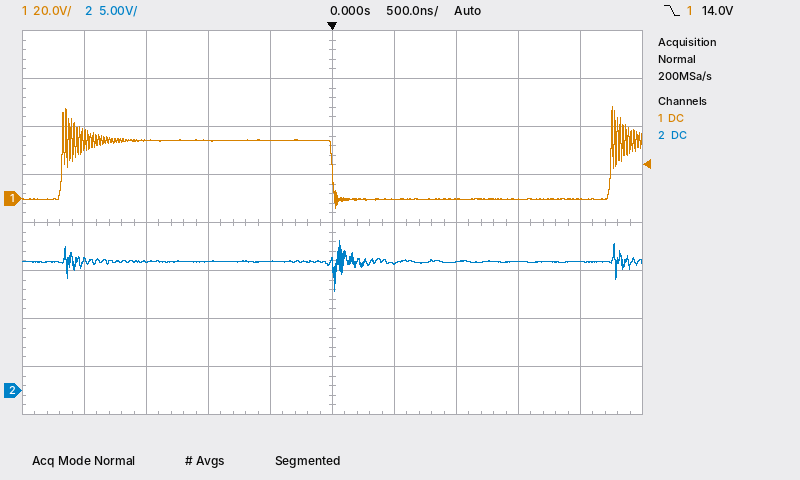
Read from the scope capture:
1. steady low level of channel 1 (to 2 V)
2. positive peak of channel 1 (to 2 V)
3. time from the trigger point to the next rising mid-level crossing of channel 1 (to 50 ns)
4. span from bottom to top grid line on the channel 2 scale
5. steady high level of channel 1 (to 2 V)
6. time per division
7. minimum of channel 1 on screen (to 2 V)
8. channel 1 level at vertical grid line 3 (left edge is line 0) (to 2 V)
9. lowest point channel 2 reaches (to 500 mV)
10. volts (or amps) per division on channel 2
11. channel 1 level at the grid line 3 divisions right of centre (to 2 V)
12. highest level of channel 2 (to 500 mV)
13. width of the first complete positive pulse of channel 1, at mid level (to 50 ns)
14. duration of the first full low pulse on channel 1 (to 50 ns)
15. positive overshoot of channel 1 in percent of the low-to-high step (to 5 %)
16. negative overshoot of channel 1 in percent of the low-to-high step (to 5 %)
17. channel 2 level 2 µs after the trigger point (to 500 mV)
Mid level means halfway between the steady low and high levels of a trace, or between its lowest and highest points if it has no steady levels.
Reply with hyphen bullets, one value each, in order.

- 0 V
- 38 V
- 2.25 µs
- 40 V
- 24 V
- 500 ns
- -4 V
- 24 V
- 10.5 V
- 5 V
- 0 V
- 15.5 V
- 2.20 µs
- 2.25 µs
- 60 %
- 15 %
- 13.5 V
